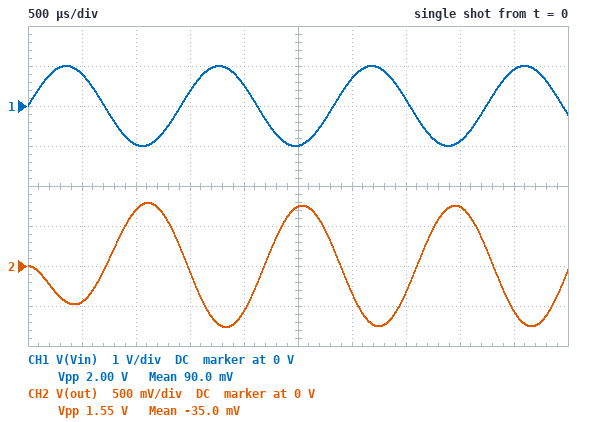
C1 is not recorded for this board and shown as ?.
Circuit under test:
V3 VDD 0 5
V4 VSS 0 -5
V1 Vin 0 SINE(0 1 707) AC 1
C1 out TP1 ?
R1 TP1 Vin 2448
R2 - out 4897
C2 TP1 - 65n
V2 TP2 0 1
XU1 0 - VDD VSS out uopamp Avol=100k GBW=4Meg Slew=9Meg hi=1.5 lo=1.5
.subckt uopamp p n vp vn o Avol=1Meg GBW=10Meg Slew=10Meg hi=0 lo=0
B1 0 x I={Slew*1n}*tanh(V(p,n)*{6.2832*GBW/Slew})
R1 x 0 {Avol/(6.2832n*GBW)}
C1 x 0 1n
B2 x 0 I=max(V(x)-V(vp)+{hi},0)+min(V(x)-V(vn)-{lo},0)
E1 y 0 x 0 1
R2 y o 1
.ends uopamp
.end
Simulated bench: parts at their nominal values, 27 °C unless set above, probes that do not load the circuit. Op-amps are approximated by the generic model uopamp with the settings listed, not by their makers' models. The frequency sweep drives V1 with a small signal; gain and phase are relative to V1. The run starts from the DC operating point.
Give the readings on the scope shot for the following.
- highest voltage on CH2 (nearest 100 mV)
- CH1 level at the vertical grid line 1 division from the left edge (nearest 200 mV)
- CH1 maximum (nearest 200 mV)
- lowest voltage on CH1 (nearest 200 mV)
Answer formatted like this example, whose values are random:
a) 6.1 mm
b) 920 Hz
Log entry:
a) 800 mV
b) 800 mV
c) 1.0 V
d) -1.0 V
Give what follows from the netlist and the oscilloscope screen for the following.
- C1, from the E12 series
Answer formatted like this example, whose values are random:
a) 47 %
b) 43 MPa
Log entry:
a) 100 nF
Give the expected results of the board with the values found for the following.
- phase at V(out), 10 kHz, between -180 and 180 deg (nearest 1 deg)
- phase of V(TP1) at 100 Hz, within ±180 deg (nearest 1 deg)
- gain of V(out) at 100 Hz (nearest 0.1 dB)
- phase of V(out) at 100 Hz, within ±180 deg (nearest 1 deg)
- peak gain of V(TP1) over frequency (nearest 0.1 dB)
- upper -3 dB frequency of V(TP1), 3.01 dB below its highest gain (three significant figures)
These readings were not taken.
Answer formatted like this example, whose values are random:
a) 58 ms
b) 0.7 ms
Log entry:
a) 95 deg
b) -15 deg
c) -14.0 dB
d) -105 deg
e) 0 dB
f) 557 Hz
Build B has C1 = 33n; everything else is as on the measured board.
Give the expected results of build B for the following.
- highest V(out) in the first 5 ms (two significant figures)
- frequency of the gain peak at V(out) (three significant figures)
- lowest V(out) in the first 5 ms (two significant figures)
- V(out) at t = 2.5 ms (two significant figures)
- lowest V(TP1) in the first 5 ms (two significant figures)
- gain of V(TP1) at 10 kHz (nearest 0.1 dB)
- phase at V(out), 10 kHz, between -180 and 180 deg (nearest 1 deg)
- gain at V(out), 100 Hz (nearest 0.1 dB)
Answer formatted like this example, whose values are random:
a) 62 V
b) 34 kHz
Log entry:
a) 1.2 V
b) 992 Hz
c) -1.2 V
d) 1.0 V
e) -850 mV
f) -40.6 dB
g) 98 deg
h) -14.0 dB
